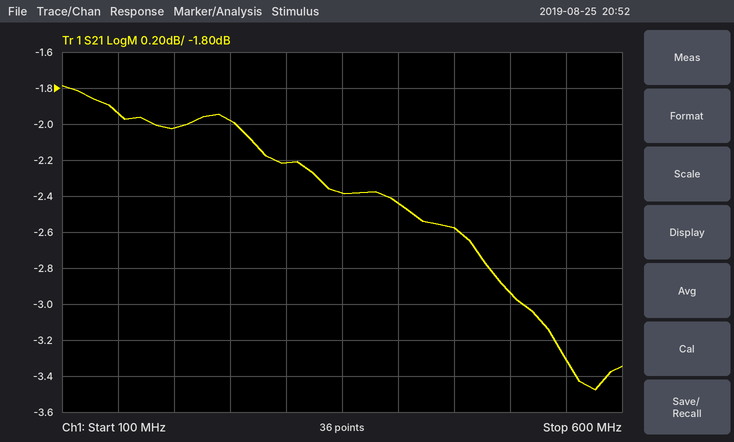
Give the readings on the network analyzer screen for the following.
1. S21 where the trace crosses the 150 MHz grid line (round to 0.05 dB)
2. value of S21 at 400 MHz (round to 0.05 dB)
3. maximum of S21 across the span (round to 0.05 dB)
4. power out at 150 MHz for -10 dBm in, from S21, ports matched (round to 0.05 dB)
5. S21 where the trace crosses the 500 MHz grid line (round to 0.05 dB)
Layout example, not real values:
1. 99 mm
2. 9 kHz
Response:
1. -1.95 dB
2. -2.45 dB
3. -1.80 dB
4. -11.95 dBm
5. -2.95 dB
